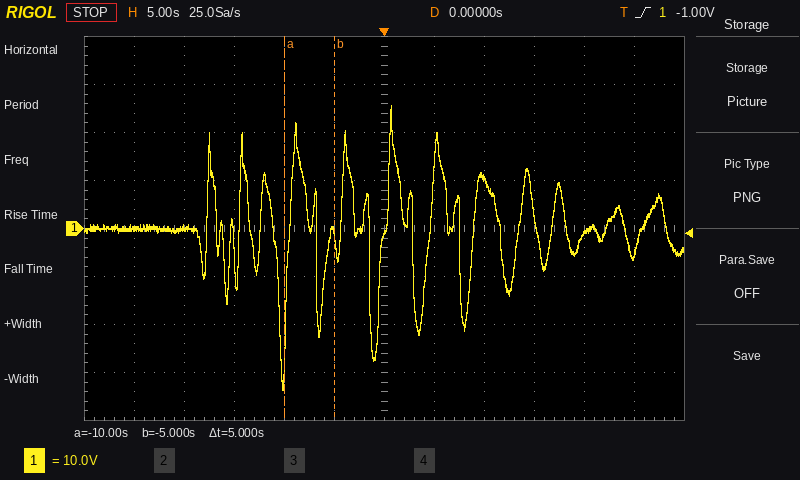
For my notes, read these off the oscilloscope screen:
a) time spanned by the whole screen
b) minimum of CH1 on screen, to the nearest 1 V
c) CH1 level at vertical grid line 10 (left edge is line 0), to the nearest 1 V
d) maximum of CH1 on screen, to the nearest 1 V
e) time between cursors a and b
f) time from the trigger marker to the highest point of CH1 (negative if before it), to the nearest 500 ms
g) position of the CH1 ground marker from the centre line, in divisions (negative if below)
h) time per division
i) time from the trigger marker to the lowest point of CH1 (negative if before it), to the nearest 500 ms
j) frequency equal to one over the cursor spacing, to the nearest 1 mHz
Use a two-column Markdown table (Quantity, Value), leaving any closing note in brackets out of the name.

| Quantity | Value |
|---|---|
| time spanned by the whole screen | 60 s |
| minimum of CH1 on screen, to the nearest 1 V | -34 V |
| CH1 level at vertical grid line 10 (left edge is line 0), to the nearest 1 V | -1 V |
| maximum of CH1 on screen, to the nearest 1 V | 26 V |
| time between cursors a and b | 5 s |
| time from the trigger marker to the highest point of CH1 (negative if before it), to the nearest 500 ms | +500 ms |
| position of the CH1 ground marker from the centre line, in divisions | 0.0 div |
| time per division | 5 s |
| time from the trigger marker to the lowest point of CH1 (negative if before it), to the nearest 500 ms | -10.0 s |
| frequency equal to one over the cursor spacing, to the nearest 1 mHz | 200 mHz |
